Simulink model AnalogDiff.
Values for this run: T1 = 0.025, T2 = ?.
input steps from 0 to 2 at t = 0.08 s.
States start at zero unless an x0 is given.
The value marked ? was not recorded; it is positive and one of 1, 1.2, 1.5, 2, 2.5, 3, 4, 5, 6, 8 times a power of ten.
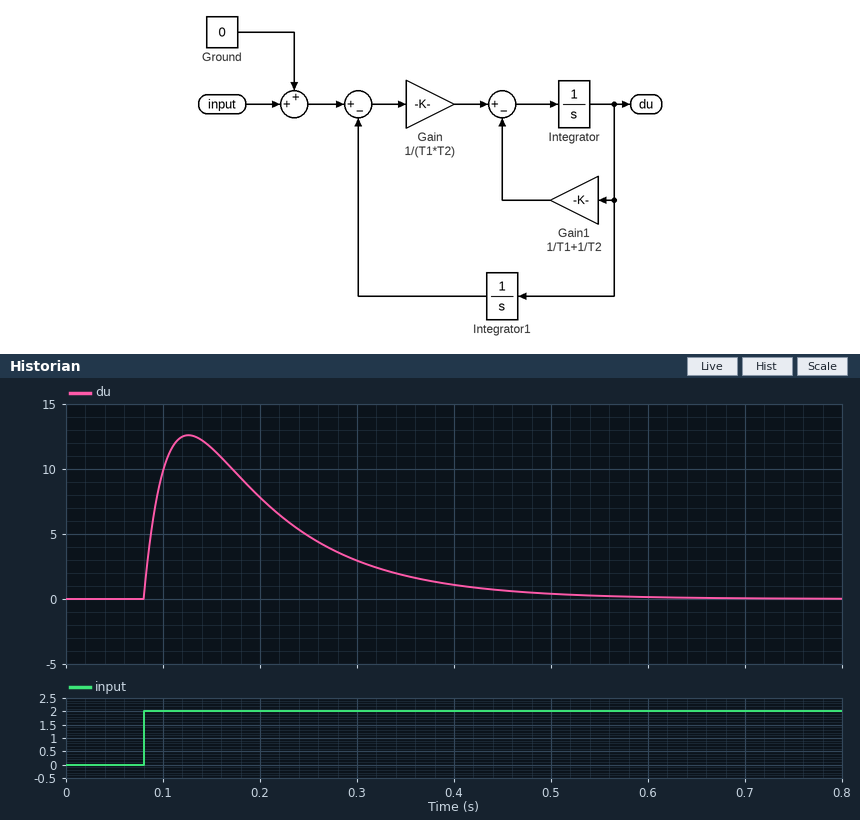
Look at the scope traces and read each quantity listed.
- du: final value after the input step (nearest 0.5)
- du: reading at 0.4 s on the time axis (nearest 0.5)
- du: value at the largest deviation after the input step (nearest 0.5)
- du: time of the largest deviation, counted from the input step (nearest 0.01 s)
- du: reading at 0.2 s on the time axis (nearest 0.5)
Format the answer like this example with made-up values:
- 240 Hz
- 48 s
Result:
- 0.0
- 1.0
- 12.5
- 0.05 s
- 8.0
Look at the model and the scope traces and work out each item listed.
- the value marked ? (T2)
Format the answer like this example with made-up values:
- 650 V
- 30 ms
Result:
- 0.1
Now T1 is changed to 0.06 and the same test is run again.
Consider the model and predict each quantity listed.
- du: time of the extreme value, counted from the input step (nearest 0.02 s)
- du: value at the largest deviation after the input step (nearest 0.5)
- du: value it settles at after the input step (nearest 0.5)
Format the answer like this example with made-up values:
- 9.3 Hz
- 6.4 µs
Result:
- 0.08 s
- 9.5
- 0.0
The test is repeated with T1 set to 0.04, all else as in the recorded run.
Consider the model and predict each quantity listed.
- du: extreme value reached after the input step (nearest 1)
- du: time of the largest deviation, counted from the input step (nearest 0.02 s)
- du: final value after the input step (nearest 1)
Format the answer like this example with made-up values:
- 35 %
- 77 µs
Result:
- 11
- 0.06 s
- 0
